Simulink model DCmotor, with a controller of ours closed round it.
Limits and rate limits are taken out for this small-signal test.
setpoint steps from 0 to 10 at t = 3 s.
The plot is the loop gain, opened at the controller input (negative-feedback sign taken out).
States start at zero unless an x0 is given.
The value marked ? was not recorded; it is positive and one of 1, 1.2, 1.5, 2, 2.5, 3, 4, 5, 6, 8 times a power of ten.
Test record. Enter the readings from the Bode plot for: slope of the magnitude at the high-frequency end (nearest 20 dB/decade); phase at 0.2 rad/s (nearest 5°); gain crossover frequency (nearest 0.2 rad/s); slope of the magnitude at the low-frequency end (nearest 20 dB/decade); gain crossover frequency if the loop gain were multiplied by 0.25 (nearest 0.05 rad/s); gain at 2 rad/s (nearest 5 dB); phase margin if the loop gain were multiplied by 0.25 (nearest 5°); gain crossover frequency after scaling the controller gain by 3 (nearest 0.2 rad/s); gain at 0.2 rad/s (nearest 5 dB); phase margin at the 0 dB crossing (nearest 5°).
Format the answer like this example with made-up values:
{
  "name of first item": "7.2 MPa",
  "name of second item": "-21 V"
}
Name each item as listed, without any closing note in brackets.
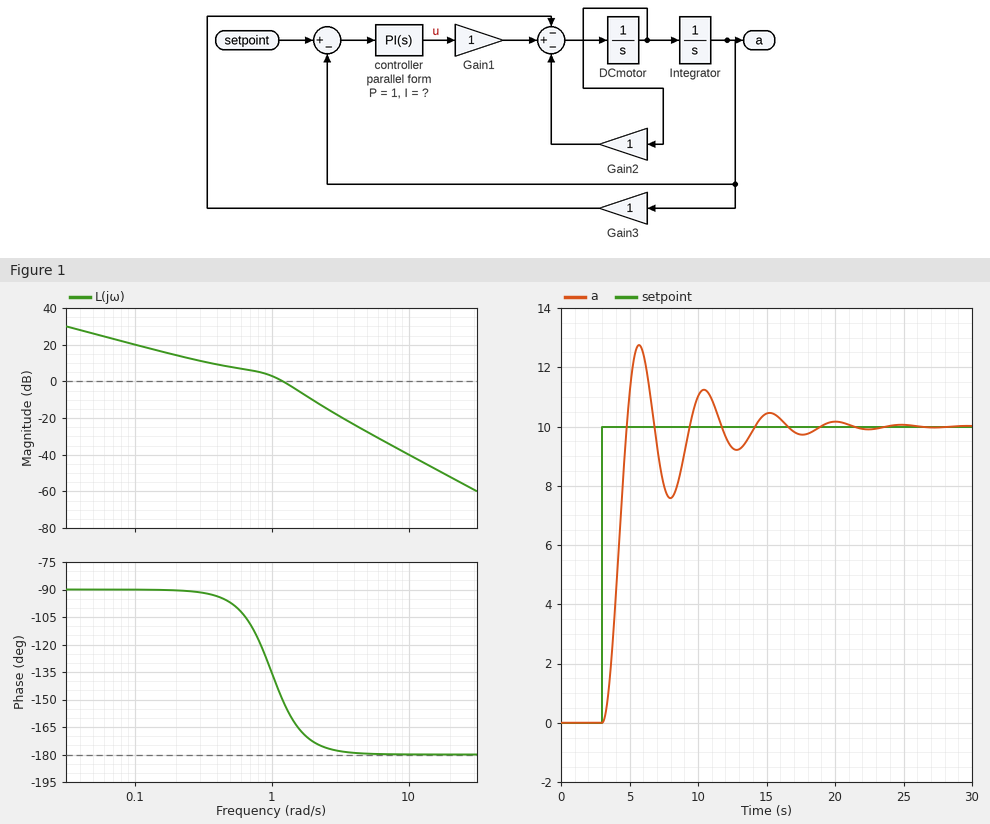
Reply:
{
  "slope of the magnitude at the high-frequency end": "-40 dB/decade",
  "phase at 0.2 rad/s": "-90°",
  "gain crossover frequency": "1.2 rad/s",
  "slope of the magnitude at the low-frequency end": "-20 dB/decade",
  "gain crossover frequency if the loop gain were multiplied by 0.25": "0.25 rad/s",
  "gain at 2 rad/s": "-10 dB",
  "phase margin if the loop gain were multiplied by 0.25": "90°",
  "gain crossover frequency after scaling the controller gain by 3": "2.0 rad/s",
  "gain at 0.2 rad/s": "15 dB",
  "phase margin at the 0 dB crossing": "30°"
}
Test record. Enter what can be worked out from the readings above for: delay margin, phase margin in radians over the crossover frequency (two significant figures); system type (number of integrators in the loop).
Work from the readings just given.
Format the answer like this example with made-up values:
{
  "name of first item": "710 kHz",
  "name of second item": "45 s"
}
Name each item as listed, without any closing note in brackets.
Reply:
{
  "delay margin, phase margin in radians over the crossover frequency": "0.44 s",
  "system type": "1"
}
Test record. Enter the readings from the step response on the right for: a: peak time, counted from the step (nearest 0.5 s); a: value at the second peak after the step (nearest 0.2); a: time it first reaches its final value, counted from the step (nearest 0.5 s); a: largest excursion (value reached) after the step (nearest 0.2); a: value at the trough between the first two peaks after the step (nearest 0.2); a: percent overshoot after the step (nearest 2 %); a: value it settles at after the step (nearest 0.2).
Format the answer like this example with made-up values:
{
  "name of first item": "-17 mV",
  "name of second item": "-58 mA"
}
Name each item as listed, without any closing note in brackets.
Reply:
{
  "a: peak time, counted from the step": "2.5 s",
  "a: value at the second peak after the step": "11.2",
  "a: time it first reaches its final value, counted from the step": "2.0 s",
  "a: largest excursion (value reached) after the step": "12.8",
  "a: value at the trough between the first two peaks after the step": "7.6",
  "a: percent overshoot after the step": "28 %",
  "a: value it settles at after the step": "10.0"
}
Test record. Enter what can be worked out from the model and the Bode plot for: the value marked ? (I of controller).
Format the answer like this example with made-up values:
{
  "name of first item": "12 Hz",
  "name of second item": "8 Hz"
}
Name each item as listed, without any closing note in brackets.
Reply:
{
  "the value marked ?": "1"
}
